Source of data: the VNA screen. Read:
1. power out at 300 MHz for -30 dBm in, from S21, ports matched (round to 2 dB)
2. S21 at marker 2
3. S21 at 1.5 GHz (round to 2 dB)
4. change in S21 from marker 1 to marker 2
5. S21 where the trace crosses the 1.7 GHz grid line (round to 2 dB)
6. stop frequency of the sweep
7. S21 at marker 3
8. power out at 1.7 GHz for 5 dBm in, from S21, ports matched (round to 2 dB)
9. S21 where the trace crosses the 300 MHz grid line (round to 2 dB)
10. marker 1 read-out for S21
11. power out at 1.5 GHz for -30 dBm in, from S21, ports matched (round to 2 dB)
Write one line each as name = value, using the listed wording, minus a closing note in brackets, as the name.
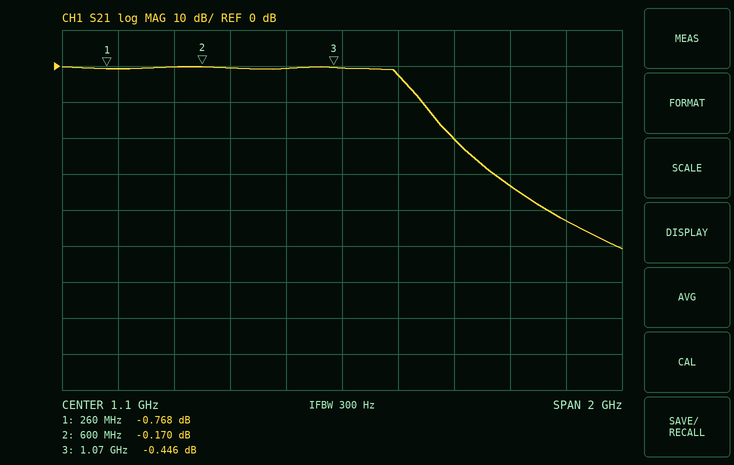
power out at 300 MHz for -30 dBm in, from S21, ports matched = -30 dBm
S21 at marker 2 = -0.170 dB
S21 at 1.5 GHz = -20 dB
change in S21 from marker 1 to marker 2 = 0.598 dB
S21 where the trace crosses the 1.7 GHz grid line = -34 dB
stop frequency of the sweep = 2.1 GHz
S21 at marker 3 = -0.446 dB
power out at 1.7 GHz for 5 dBm in, from S21, ports matched = -28 dBm
S21 where the trace crosses the 300 MHz grid line = 0 dB
marker 1 read-out for S21 = -0.768 dB
power out at 1.5 GHz for -30 dBm in, from S21, ports matched = -50 dBm
